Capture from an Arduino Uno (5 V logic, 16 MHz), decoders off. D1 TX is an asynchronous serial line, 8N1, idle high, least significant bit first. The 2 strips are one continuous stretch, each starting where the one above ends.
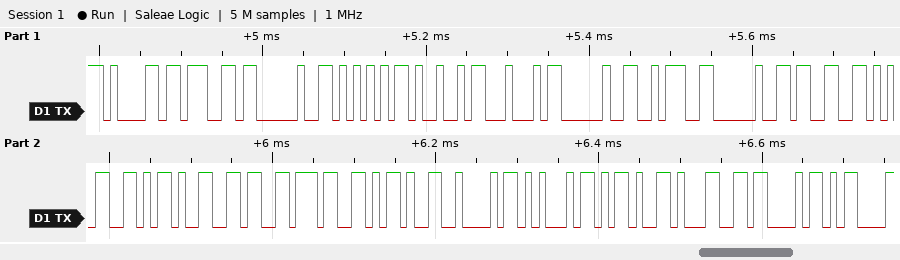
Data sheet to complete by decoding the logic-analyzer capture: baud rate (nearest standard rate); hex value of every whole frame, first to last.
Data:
115200 baud
0x61 0x67 0x20 0x55 0x49 0x44 0x20 0x3A 0x20 0x33 0x35 0x2D 0x36 0x37 0x2D 0x42 0x45 0x2D 0x31 0x43 0x0D
